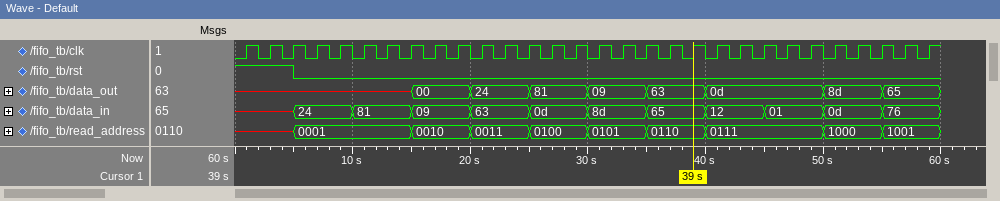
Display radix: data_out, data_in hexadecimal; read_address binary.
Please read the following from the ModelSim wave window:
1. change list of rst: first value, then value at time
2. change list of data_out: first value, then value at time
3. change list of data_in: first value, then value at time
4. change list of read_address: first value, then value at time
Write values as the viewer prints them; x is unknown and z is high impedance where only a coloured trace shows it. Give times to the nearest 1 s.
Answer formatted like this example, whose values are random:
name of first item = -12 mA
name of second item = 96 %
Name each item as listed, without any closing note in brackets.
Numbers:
change list of rst: first value, then value at time = 1, 0 at 5 s
change list of data_out: first value, then value at time = x, 00 at 15 s, 24 at 20 s, 81 at 25 s, 09 at 30 s, 63 at 35 s, 0d at 40 s, 8d at 50 s, 65 at 55 s
change list of data_in: first value, then value at time = x, 24 at 5 s, 81 at 10 s, 09 at 15 s, 63 at 20 s, 0d at 25 s, 8d at 30 s, 65 at 35 s, 12 at 40 s, 01 at 45 s, 0d at 50 s, 76 at 55 s
change list of read_address: first value, then value at time = x, 0001 at 5 s, 0010 at 15 s, 0011 at 20 s, 0100 at 25 s, 0101 at 30 s, 0110 at 35 s, 0111 at 40 s, 1000 at 50 s, 1001 at 55 s
